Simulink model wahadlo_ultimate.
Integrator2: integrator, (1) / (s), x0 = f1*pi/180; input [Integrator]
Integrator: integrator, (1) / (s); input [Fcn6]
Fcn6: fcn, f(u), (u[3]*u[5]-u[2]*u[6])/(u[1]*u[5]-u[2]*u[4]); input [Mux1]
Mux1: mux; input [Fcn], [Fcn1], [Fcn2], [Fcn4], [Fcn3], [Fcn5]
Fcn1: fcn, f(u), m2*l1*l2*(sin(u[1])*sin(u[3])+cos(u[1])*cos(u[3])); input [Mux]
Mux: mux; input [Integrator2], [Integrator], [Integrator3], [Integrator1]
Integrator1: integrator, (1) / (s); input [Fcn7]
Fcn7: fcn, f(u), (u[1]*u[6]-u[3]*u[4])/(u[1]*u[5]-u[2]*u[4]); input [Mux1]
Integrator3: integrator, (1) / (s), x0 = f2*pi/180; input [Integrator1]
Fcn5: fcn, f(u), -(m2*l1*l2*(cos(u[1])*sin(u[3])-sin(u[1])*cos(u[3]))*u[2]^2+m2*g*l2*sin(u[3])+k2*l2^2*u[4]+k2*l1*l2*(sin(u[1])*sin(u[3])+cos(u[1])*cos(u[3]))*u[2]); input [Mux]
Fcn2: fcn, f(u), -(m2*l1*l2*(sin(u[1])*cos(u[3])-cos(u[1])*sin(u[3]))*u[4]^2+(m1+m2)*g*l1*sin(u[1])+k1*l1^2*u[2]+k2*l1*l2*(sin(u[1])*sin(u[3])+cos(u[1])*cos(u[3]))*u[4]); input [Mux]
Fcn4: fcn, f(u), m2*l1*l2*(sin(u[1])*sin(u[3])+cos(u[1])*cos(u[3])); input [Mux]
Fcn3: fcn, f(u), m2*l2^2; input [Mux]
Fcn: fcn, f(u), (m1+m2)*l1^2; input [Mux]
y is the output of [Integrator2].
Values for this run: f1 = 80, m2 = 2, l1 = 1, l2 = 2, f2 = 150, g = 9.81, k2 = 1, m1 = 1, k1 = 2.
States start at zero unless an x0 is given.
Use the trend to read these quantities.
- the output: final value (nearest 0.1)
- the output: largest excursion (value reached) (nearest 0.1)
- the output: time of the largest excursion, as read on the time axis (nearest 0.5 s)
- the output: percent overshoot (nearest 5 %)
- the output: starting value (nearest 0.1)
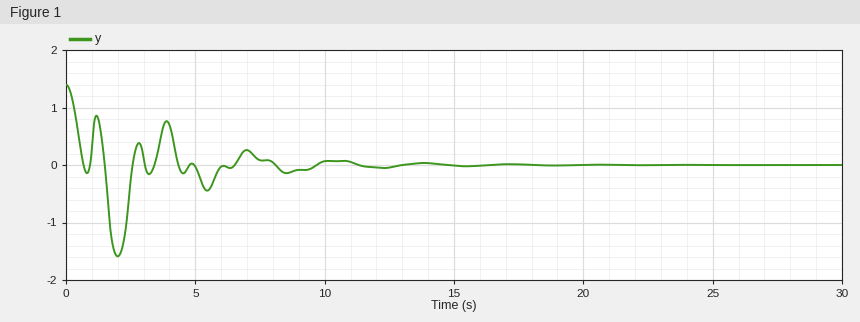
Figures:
0.0
-1.6
2.0 s
115 %
1.4
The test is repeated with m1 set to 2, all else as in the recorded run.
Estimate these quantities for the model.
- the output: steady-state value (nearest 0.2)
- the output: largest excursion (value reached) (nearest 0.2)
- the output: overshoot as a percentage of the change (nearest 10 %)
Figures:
0.0
-1.2
90 %
